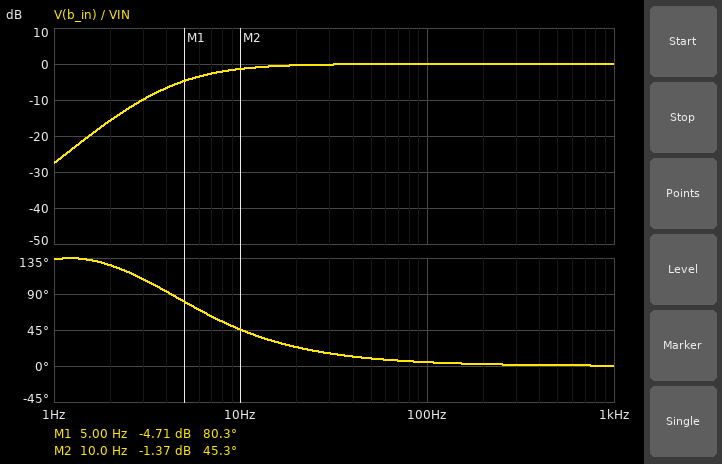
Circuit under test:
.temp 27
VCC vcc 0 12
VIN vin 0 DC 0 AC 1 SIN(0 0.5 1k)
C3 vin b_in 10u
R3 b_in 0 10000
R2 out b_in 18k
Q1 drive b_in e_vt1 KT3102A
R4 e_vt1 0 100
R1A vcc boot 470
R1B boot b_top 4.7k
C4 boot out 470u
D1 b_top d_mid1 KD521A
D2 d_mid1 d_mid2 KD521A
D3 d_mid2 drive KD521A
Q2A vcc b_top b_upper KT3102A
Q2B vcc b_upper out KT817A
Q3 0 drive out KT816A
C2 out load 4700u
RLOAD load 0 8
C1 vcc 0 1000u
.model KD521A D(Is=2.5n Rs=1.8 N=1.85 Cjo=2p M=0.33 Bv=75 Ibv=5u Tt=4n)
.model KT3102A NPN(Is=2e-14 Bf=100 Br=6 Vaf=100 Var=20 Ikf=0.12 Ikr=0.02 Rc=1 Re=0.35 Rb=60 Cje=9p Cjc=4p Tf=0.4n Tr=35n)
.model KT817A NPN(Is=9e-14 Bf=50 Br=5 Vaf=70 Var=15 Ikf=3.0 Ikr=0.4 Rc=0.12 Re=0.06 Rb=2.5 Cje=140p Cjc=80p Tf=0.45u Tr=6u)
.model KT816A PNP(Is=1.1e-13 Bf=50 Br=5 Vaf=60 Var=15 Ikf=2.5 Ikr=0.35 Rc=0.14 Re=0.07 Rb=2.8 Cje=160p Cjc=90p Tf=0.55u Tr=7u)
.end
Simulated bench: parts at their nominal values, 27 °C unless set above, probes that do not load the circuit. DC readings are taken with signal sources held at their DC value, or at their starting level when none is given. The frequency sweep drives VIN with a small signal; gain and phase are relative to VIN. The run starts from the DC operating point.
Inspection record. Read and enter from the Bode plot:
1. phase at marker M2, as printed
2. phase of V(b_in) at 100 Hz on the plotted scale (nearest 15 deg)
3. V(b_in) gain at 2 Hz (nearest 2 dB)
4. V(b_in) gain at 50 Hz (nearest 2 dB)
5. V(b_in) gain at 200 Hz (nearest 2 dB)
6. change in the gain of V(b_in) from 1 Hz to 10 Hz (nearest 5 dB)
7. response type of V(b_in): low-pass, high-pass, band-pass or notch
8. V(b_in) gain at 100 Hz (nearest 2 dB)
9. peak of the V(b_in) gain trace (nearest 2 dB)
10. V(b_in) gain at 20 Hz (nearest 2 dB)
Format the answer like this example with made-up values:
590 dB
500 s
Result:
45.3 deg
0 deg
-16 dB
0 dB
0 dB
25 dB
high-pass
0 dB
0 dB
0 dB
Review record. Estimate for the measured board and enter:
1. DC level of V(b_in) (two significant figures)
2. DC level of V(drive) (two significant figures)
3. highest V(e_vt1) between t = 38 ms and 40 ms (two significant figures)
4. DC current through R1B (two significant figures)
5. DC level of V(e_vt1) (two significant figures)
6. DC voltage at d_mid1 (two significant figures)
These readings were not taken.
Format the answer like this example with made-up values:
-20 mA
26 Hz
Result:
840 mV
2.0 V
910 mV
1.6 mA
180 mV
3.3 V
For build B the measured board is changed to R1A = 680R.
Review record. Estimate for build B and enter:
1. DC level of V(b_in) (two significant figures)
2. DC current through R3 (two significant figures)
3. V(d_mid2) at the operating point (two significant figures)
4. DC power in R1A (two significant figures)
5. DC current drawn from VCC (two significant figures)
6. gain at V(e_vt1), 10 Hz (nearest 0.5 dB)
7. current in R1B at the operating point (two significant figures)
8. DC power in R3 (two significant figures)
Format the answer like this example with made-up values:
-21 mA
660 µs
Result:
830 mV
83 µA
2.6 V
1.5 mW
14 mA
-2.5 dB
1.5 mA
69 µW
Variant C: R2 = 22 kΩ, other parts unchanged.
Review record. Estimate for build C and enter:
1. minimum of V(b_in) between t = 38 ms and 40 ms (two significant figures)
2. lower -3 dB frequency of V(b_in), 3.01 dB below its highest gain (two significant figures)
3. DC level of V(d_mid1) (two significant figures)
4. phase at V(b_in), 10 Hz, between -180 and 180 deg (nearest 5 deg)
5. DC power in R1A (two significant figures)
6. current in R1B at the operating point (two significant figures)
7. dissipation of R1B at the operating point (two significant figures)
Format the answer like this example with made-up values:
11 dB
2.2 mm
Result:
600 mV
5.7 Hz
3.7 V
40 deg
1.0 mW
1.5 mA
10 mW
